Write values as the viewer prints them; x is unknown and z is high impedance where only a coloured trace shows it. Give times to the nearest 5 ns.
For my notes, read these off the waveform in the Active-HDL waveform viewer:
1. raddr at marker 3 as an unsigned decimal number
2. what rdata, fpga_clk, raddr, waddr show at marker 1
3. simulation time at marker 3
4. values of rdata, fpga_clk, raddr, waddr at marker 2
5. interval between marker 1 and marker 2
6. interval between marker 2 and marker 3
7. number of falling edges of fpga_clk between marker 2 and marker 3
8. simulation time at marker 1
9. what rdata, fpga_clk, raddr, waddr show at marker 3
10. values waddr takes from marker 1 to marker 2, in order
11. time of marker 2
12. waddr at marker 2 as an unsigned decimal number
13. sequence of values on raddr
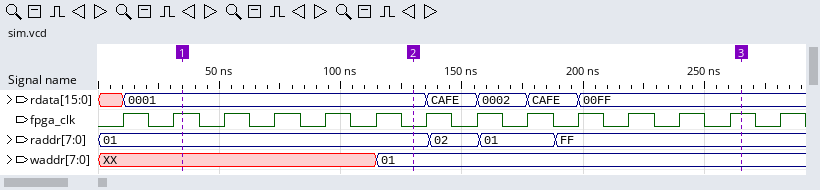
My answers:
255
rdata=0001, fpga_clk=1, raddr=01, waddr=XX
265 ns
rdata=0001, fpga_clk=0, raddr=01, waddr=01
95 ns
135 ns
6
35 ns
rdata=00FF, fpga_clk=1, raddr=FF, waddr=01
XX, 01
130 ns
1
01, 02, 01, FF
